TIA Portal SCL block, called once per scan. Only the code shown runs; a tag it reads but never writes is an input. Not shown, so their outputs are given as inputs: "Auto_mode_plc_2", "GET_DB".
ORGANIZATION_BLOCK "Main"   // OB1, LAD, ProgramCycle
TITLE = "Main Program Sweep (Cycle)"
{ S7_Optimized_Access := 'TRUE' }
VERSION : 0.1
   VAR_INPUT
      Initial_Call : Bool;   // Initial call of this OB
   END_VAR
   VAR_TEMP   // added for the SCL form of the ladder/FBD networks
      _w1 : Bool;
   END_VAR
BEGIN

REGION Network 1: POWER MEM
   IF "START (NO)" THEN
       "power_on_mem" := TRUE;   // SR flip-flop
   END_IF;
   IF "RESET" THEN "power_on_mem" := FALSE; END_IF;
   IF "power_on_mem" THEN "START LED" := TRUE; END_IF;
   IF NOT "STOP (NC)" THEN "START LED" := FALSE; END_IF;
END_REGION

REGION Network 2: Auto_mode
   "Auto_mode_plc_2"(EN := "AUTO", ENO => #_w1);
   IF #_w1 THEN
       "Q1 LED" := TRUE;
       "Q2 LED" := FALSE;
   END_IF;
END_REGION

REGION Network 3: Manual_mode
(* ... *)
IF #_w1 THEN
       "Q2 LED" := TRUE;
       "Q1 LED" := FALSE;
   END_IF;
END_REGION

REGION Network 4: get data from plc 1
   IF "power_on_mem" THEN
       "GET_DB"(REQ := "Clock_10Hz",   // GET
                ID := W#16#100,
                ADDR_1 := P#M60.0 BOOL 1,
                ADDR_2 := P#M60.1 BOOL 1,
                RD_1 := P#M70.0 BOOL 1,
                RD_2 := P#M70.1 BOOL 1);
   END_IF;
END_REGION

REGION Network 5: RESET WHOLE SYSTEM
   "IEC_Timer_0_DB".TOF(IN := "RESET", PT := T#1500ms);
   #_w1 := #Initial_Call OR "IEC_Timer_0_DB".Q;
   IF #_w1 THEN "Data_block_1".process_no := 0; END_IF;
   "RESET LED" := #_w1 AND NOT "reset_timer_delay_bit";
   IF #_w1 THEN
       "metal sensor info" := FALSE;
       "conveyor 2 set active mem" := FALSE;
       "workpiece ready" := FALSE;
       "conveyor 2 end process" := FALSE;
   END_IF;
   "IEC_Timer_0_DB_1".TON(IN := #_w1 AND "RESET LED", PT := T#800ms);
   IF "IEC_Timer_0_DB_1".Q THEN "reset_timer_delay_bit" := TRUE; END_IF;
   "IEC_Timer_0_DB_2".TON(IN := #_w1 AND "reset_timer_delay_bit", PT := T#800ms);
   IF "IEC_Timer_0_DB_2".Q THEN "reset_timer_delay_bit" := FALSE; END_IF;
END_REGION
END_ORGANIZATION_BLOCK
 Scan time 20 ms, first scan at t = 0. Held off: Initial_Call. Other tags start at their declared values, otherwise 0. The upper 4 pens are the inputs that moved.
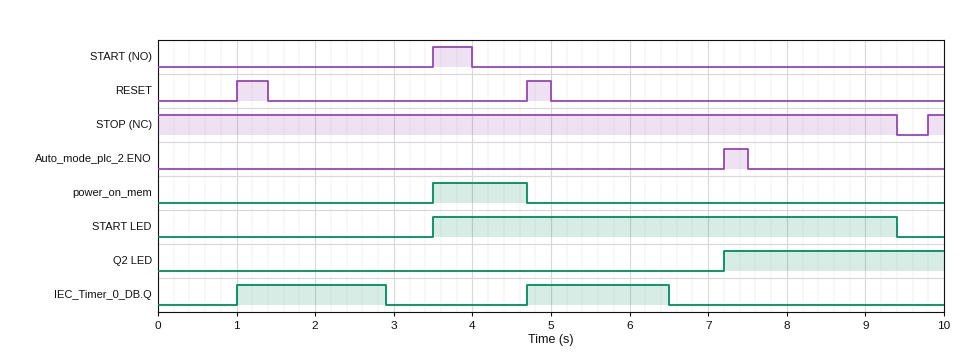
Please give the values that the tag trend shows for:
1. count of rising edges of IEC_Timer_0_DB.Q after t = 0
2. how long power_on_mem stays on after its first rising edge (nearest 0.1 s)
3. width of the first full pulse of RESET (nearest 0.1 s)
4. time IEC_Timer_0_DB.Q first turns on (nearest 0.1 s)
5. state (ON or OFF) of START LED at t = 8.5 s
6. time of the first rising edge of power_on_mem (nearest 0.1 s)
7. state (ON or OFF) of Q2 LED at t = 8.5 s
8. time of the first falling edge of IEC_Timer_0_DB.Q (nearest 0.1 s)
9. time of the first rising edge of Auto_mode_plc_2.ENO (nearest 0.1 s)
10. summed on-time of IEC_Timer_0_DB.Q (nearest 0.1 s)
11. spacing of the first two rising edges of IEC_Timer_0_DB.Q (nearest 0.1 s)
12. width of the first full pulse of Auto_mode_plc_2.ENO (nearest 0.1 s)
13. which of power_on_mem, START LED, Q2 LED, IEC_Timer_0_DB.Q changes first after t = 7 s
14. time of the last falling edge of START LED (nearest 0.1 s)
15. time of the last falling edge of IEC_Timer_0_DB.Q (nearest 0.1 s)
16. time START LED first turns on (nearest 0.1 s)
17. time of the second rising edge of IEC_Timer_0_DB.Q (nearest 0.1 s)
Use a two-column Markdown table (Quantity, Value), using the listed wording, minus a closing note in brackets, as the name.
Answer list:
| Quantity | Value |
|---|---|
| count of rising edges of IEC_Timer_0_DB.Q after t = 0 | 2 |
| how long power_on_mem stays on after its first rising edge | 1.2 s |
| width of the first full pulse of RESET | 0.4 s |
| time IEC_Timer_0_DB.Q first turns on | 1.0 s |
| state (ON or OFF) of START LED at t = 8.5 s | ON |
| time of the first rising edge of power_on_mem | 3.5 s |
| state (ON or OFF) of Q2 LED at t = 8.5 s | ON |
| time of the first falling edge of IEC_Timer_0_DB.Q | 2.9 s |
| time of the first rising edge of Auto_mode_plc_2.ENO | 7.2 s |
| summed on-time of IEC_Timer_0_DB.Q | 3.7 s |
| spacing of the first two rising edges of IEC_Timer_0_DB.Q | 3.7 s |
| width of the first full pulse of Auto_mode_plc_2.ENO | 0.3 s |
| which of power_on_mem, START LED, Q2 LED, IEC_Timer_0_DB.Q changes first after t = 7 s | Q2 LED |
| time of the last falling edge of START LED | 9.4 s |
| time of the last falling edge of IEC_Timer_0_DB.Q | 6.5 s |
| time START LED first turns on | 3.5 s |
| time of the second rising edge of IEC_Timer_0_DB.Q | 4.7 s |
